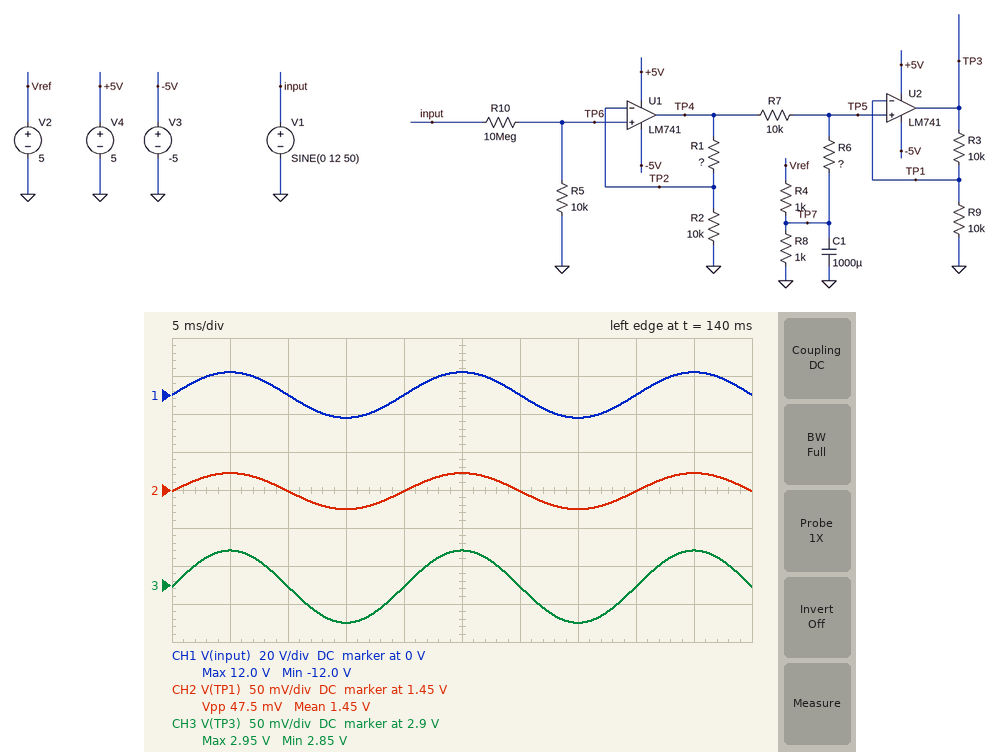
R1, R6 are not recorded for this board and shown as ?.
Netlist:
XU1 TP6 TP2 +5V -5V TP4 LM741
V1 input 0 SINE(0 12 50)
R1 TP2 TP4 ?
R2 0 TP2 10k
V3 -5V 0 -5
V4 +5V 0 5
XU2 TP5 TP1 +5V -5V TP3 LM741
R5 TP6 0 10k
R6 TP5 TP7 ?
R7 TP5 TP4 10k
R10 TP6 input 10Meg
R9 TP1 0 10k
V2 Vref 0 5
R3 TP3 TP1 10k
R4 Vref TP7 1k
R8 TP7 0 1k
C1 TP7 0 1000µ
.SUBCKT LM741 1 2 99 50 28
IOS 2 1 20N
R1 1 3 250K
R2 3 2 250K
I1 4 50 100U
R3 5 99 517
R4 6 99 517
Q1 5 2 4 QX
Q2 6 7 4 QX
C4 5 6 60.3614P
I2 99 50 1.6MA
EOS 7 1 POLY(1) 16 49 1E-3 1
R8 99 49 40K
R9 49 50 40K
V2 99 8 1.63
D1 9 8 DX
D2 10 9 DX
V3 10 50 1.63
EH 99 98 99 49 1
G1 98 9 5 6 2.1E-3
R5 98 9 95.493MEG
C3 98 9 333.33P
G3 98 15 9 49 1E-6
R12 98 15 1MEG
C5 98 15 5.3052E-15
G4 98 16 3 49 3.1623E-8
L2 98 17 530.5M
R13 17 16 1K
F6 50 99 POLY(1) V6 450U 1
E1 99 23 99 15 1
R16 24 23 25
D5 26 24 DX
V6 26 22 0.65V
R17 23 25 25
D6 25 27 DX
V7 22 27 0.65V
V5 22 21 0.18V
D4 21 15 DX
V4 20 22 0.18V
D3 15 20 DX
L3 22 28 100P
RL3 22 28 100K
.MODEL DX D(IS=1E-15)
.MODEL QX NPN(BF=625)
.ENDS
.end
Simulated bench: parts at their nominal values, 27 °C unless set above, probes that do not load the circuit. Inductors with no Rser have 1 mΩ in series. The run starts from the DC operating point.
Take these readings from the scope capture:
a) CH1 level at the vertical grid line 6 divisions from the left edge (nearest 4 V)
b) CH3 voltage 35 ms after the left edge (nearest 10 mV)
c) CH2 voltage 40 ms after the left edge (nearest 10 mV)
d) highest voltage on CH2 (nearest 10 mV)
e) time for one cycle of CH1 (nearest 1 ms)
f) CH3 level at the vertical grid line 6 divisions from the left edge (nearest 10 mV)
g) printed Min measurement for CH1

0 V
2.85 V
1.45 V
1.47 V
20 ms
2.90 V
-12.0 V
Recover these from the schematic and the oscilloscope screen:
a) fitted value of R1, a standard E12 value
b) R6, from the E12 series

39 kΩ
6.8 kΩ
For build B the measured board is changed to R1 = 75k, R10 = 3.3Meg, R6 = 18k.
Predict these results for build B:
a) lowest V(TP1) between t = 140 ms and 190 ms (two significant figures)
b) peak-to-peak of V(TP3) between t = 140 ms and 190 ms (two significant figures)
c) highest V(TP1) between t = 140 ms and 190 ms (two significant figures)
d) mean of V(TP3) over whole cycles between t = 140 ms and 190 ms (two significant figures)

690 mV
790 mV
1.1 V
1.8 V
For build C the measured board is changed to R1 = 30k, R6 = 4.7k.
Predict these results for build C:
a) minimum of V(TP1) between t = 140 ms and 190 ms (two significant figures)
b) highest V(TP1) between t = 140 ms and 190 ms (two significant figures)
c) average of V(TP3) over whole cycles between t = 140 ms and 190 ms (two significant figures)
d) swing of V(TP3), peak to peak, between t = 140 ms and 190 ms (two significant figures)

1.6 V
1.7 V
3.3 V
61 mV
